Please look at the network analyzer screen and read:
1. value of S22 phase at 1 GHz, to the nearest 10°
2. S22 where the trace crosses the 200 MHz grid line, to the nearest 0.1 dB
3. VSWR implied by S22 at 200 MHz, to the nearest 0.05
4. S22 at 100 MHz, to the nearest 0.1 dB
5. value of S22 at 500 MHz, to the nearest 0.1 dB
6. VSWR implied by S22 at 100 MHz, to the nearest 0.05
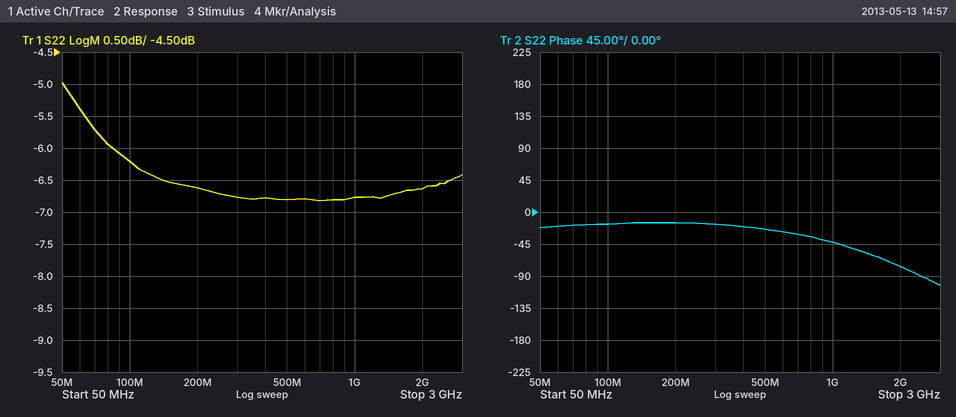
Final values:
-40°
-6.6 dB
2.75
-6.2 dB
-6.8 dB
2.90
